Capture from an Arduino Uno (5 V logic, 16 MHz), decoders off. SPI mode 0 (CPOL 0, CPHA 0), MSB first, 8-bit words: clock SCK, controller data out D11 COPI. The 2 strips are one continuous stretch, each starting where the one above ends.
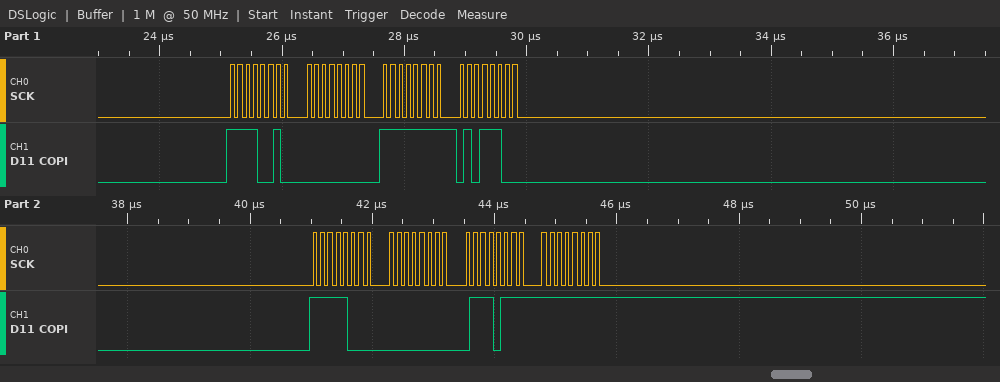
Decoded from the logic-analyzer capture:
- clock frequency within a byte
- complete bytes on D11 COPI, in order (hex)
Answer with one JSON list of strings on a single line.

["8 MHz", "F2 00 FF 5C F8 00 77 FF"]
